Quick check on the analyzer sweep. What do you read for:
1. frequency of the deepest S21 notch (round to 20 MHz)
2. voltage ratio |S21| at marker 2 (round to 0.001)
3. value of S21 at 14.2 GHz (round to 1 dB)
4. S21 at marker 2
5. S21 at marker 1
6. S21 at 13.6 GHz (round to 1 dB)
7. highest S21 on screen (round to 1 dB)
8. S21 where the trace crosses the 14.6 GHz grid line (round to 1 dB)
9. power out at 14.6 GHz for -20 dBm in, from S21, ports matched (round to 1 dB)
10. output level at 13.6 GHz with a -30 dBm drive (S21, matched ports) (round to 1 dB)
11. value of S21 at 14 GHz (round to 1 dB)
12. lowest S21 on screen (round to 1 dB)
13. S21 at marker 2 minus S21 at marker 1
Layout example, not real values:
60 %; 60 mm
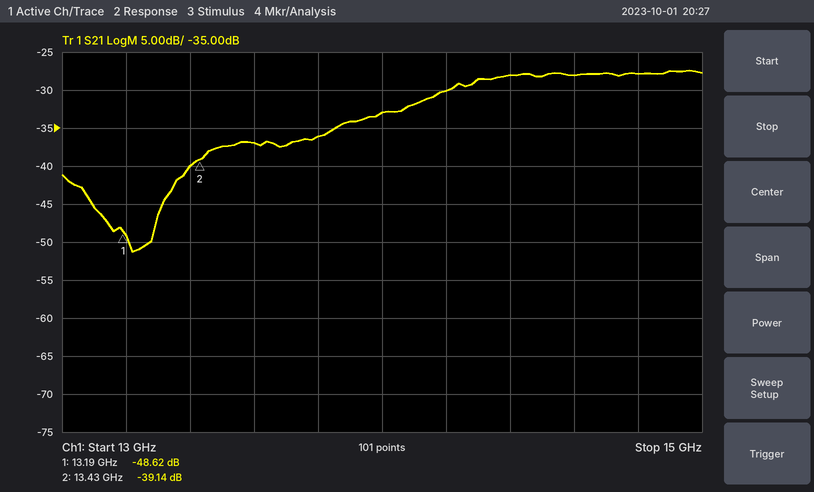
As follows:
13.22 GHz; 0.011; -30 dB; -39.14 dB; -48.62 dB; -37 dB; -27 dB; -28 dB; -48 dBm; -67 dBm; -33 dB; -51 dB; 9.48 dB
